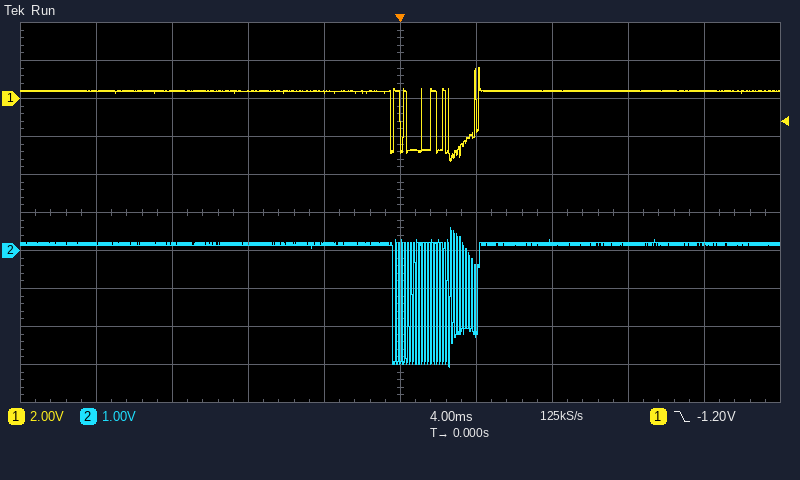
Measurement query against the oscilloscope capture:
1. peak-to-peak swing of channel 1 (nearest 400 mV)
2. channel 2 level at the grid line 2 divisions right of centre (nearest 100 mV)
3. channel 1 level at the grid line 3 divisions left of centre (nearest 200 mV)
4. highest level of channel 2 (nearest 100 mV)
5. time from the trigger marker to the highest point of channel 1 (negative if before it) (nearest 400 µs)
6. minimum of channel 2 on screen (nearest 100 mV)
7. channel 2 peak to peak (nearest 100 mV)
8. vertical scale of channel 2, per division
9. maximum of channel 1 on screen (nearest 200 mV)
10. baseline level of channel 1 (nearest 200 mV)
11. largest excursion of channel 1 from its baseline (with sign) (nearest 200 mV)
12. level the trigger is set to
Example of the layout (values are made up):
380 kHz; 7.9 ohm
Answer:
4.8 V; 200 mV; 400 mV; 600 mV; +4.0 ms; -3.1 V; 3.7 V; 1 V; 1.6 V; 400 mV; -3.8 V; -1.20 V
